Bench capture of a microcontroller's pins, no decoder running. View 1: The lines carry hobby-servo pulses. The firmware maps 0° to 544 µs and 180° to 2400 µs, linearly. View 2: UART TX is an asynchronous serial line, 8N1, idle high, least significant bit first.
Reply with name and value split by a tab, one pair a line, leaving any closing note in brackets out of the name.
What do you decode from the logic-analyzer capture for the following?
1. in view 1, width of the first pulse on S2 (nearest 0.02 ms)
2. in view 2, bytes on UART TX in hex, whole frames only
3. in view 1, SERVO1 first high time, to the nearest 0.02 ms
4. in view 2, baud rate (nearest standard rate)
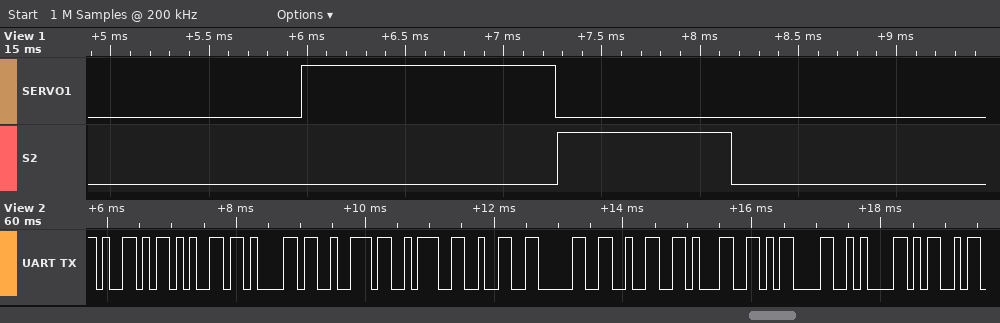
in view 1, width of the first pulse on S2	0.88 ms
in view 2, bytes on UART TX in hex, whole frames only	59 65 61 72 3A 32 30 32 31 0D 0A 4D
in view 1, SERVO1 first high time, to the nearest 0.02 ms	1.30 ms
in view 2, baud rate	9600 baud
